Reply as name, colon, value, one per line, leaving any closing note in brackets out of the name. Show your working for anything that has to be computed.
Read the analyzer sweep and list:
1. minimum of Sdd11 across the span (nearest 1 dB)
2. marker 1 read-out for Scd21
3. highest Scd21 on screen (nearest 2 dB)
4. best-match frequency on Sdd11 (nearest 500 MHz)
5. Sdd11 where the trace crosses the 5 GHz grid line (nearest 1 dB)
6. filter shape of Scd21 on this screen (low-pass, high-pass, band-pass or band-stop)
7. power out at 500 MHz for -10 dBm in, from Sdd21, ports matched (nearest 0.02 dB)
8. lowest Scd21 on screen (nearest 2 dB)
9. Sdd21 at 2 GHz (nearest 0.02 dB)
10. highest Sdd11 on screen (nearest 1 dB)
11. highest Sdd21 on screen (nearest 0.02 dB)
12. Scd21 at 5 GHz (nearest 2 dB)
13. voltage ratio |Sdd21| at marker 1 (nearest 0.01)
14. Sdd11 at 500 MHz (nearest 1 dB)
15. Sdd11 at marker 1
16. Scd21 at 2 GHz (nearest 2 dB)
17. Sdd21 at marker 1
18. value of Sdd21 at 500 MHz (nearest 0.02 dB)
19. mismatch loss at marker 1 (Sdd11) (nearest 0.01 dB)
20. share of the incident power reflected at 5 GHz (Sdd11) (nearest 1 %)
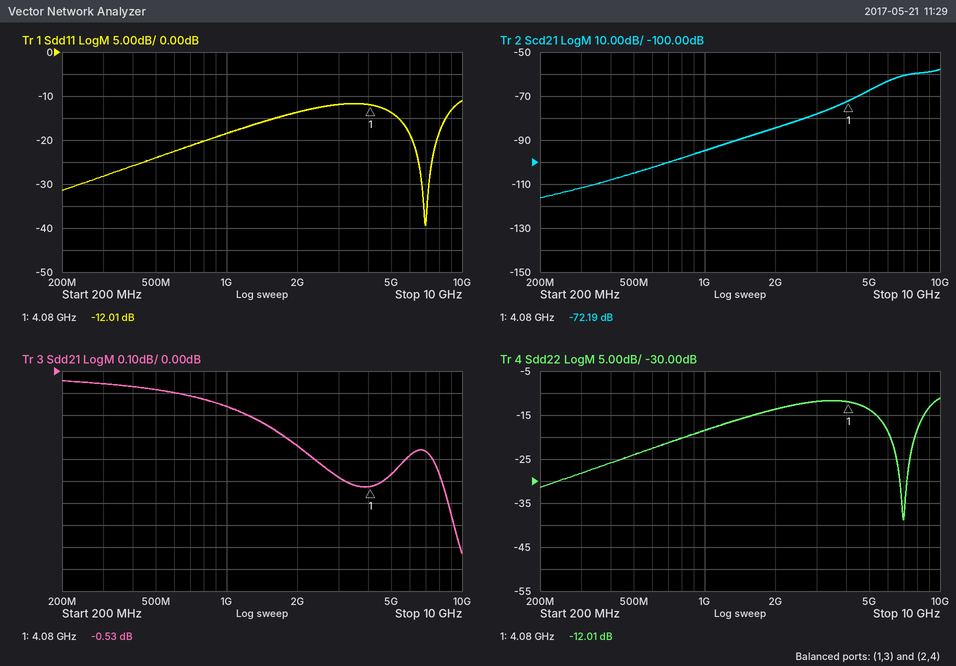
minimum of Sdd11 across the span: -39 dB
marker 1 read-out for Scd21: -72.19 dB
highest Scd21 on screen: -58 dB
best-match frequency on Sdd11: 7.0 GHz
Sdd11 where the trace crosses the 5 GHz grid line: -14 dB
filter shape of Scd21 on this screen: high-pass
power out at 500 MHz for -10 dBm in, from Sdd21, ports matched: -10 dBm + (-0.08 dB) = -10.08 dBm
lowest Scd21 on screen: -116 dB
Sdd21 at 2 GHz: -0.34 dB
highest Sdd11 on screen: -11 dB
highest Sdd21 on screen: -0.04 dB
Scd21 at 5 GHz: -68 dB
voltage ratio |Sdd21| at marker 1: 10^(-0.53/20) ≈ 0.94
Sdd11 at 500 MHz: -24 dB
Sdd11 at marker 1: -12.01 dB
Scd21 at 2 GHz: -84 dB
Sdd21 at marker 1: -0.53 dB
value of Sdd21 at 500 MHz: -0.08 dB
mismatch loss at marker 1 (Sdd11): −10 log10(1 − 10^(-12.01/10)) ≈ 0.28 dB
share of the incident power reflected at 5 GHz (Sdd11): 10^(-14/10) ≈ 4 %
